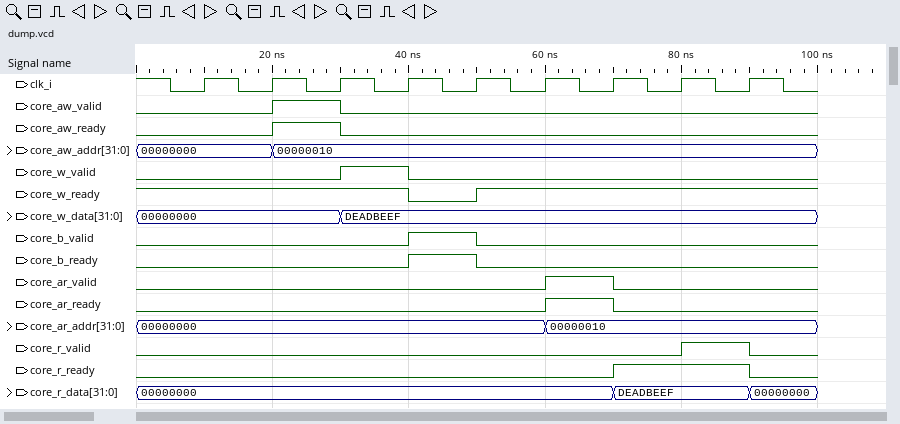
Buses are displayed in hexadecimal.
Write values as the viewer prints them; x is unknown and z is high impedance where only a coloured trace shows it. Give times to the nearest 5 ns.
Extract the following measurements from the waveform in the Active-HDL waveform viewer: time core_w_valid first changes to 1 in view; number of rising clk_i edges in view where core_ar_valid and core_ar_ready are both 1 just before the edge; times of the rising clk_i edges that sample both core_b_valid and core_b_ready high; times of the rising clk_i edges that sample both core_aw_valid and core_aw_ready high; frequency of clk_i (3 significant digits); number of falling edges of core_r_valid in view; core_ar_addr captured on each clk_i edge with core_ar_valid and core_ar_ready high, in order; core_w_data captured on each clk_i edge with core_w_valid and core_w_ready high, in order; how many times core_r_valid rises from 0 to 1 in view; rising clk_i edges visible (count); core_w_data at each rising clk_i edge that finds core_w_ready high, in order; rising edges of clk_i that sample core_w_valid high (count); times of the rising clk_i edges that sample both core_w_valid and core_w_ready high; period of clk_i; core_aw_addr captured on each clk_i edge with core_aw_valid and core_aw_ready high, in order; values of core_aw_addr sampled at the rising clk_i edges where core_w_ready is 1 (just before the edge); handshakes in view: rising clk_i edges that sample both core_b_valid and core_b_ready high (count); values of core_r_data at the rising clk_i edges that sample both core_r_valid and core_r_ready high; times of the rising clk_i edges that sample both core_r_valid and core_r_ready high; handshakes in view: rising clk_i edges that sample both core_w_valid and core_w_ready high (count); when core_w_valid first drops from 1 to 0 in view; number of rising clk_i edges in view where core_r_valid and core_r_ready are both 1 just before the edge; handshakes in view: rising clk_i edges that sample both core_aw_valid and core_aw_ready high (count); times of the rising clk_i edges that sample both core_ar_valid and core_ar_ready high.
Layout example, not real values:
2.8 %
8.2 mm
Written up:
30 ns
1
50 ns
30 ns
100 MHz
1
00000010
DEADBEEF
1
9
00000000, 00000000, 00000000, DEADBEEF, DEADBEEF, DEADBEEF, DEADBEEF, DEADBEEF
1
40 ns
10 ns
00000010
00000000, 00000000, 00000010, 00000010, 00000010, 00000010, 00000010, 00000010
1
DEADBEEF
90 ns
1
40 ns
1
1
70 ns
